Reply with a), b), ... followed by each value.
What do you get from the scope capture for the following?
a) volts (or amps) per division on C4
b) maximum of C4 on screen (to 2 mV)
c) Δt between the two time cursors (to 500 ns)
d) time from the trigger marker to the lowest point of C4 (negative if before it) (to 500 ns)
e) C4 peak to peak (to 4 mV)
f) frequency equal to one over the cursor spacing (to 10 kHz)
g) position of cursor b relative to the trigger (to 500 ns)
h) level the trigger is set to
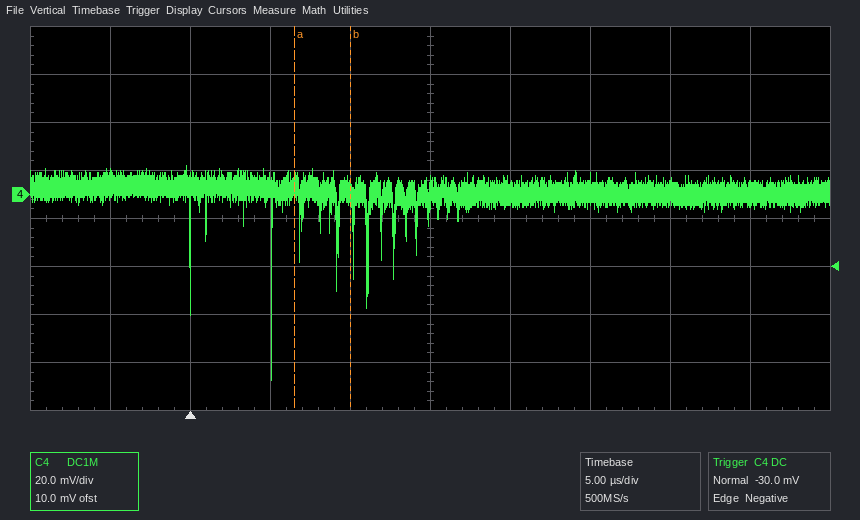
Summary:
a) 20 mV
b) 12 mV
c) 3.5 µs
d) +5.0 µs
e) 88 mV
f) 290 kHz
g) +10.0 µs
h) -30.0 mV
